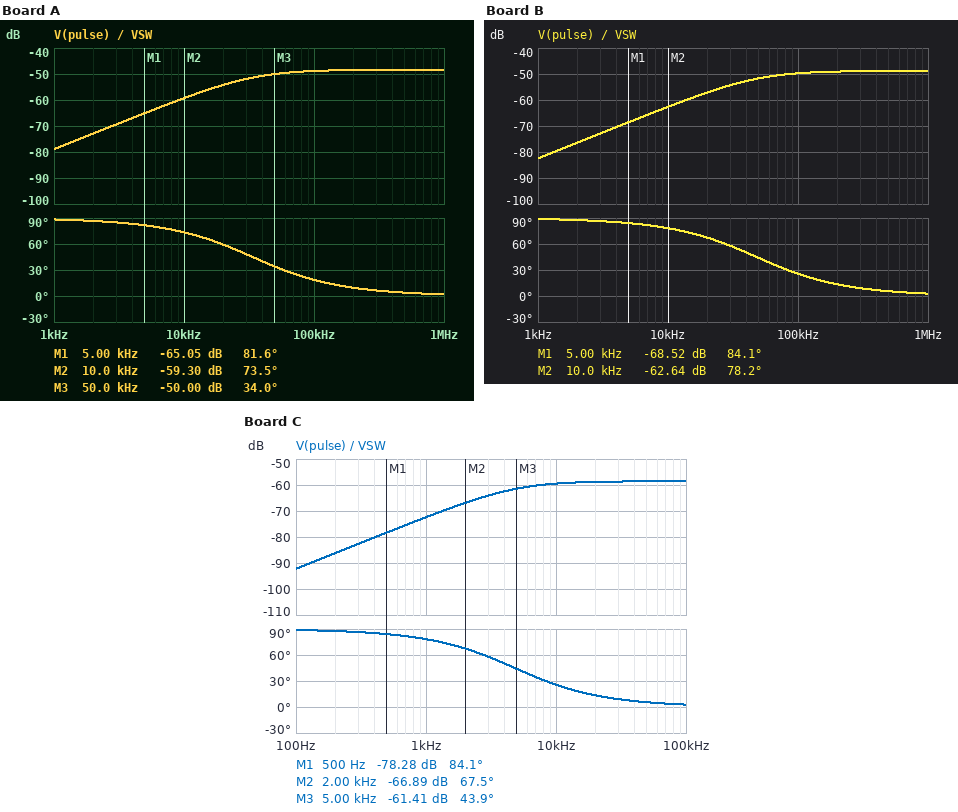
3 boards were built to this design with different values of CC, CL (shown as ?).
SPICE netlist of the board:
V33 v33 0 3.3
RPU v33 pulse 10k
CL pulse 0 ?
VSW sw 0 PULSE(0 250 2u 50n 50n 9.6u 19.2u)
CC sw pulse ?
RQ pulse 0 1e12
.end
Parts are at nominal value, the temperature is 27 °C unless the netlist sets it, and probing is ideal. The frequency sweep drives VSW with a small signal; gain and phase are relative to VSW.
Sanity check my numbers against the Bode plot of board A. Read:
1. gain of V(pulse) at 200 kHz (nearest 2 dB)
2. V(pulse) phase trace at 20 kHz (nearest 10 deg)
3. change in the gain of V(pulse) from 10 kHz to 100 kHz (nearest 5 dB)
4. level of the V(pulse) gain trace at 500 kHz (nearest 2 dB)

-48 dB
60 deg
10 dB
-48 dB
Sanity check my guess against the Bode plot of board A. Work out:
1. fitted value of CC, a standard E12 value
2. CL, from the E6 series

1.8 pF
470 pF
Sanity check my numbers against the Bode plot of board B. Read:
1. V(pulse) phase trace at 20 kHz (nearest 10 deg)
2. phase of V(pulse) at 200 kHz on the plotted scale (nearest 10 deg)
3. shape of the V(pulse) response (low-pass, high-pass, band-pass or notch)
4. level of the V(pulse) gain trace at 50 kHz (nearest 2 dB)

70 deg
10 deg
high-pass
-52 dB
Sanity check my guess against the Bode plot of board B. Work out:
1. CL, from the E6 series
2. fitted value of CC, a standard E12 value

330 pF
1.2 pF
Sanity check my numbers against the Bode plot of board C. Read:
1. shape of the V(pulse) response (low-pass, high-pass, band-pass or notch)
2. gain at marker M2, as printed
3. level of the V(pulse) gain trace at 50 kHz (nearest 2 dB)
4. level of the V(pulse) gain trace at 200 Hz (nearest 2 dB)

high-pass
-66.89 dB
-58 dB
-86 dB
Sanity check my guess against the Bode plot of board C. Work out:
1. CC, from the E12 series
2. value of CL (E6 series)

3.9 pF
3.3 nF
